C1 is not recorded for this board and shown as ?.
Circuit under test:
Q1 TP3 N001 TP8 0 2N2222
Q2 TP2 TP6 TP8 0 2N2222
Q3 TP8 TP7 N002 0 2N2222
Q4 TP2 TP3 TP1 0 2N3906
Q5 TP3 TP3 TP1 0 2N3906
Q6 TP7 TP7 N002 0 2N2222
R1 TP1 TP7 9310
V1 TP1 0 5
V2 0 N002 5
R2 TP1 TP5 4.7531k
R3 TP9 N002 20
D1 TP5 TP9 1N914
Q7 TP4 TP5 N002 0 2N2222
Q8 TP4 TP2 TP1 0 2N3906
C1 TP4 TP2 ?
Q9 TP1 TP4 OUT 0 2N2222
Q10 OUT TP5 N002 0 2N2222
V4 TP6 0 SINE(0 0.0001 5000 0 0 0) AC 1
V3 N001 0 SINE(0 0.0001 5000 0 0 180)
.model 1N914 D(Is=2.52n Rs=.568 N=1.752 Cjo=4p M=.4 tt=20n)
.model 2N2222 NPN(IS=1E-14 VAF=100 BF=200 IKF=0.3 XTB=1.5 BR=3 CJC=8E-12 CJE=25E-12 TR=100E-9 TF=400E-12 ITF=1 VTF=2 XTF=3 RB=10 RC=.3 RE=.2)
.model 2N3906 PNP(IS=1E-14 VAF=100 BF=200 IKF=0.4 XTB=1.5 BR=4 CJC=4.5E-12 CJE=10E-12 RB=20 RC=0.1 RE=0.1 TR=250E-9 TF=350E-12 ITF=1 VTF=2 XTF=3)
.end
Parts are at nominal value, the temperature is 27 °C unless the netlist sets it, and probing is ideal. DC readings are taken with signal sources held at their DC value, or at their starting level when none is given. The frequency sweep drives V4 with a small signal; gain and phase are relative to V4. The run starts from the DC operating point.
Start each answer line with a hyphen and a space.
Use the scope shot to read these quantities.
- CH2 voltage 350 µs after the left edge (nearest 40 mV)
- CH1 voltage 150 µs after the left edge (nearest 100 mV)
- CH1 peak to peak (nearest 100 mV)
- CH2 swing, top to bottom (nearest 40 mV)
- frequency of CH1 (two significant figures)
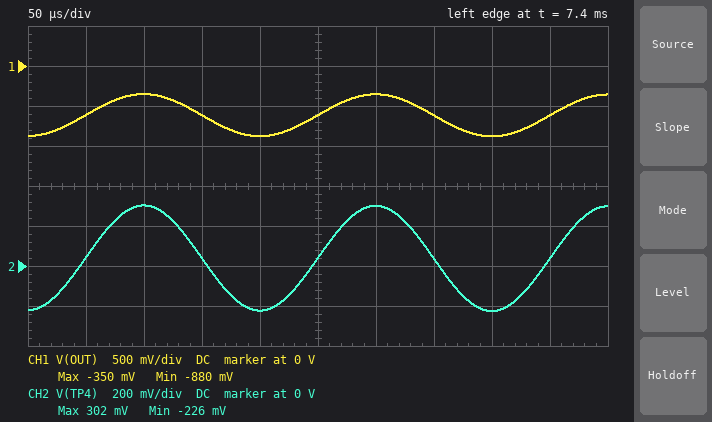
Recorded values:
- 40 mV
- -600 mV
- 500 mV
- 520 mV
- 5.0 kHz
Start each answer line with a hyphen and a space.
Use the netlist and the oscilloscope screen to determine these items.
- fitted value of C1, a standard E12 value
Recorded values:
- 470 pF
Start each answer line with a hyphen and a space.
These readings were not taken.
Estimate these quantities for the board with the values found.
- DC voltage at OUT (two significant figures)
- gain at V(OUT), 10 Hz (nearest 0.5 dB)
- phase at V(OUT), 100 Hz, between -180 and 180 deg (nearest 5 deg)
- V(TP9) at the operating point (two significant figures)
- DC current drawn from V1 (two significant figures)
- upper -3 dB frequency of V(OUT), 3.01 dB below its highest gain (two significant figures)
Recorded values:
- -670 mV
- 105.5 dB
- -70 deg
- -5.0 V
- 6.0 mA
- 33 Hz
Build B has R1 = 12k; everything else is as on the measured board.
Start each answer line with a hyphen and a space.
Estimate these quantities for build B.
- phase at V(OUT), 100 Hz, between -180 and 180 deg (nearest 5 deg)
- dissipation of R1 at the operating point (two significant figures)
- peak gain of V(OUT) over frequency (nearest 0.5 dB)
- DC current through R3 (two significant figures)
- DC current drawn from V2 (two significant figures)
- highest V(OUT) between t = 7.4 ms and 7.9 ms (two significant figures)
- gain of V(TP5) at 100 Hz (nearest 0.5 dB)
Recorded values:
- 0 deg
- 7.3 mW
- 56.5 dB
- 1.9 mA
- 4.8 mA
- -4.9 V
- 39.5 dB
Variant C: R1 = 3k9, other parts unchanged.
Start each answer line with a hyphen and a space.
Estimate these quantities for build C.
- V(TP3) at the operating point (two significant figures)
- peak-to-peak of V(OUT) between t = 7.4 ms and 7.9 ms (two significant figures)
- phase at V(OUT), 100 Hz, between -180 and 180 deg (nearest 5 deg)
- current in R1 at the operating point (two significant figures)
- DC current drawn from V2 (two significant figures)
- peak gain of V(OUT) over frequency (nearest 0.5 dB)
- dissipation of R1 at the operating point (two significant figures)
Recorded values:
- 4.3 V
- 240 mV
- 0 deg
- 2.4 mA
- 8.9 mA
- 44.5 dB
- 22 mW
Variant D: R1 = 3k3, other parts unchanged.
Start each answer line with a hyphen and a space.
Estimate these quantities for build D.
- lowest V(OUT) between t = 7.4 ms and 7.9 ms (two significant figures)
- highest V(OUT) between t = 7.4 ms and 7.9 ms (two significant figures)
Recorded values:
- 4.1 V
- 4.3 V
